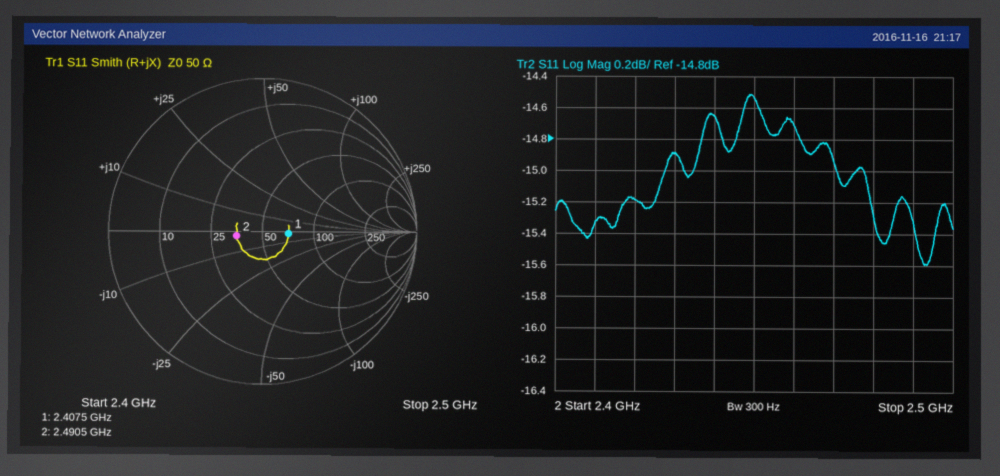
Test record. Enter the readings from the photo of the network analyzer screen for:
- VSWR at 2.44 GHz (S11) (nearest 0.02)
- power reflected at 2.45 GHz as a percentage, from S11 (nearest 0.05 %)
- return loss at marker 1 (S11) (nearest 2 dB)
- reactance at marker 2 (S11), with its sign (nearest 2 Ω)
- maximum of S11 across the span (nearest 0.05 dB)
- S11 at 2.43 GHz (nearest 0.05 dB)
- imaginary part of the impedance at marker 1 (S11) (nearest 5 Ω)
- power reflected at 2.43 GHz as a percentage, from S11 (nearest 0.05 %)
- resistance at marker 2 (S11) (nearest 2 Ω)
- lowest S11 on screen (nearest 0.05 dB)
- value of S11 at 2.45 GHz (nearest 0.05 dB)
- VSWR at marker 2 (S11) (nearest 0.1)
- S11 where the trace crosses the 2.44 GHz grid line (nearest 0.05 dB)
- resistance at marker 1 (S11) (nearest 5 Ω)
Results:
1.46
3.50 %
16 dB
-2 Ω
-14.50 dB
-14.90 dB
0 Ω
3.25 %
36 Ω
-15.60 dB
-14.55 dB
1.4
-14.65 dB
70 Ω
